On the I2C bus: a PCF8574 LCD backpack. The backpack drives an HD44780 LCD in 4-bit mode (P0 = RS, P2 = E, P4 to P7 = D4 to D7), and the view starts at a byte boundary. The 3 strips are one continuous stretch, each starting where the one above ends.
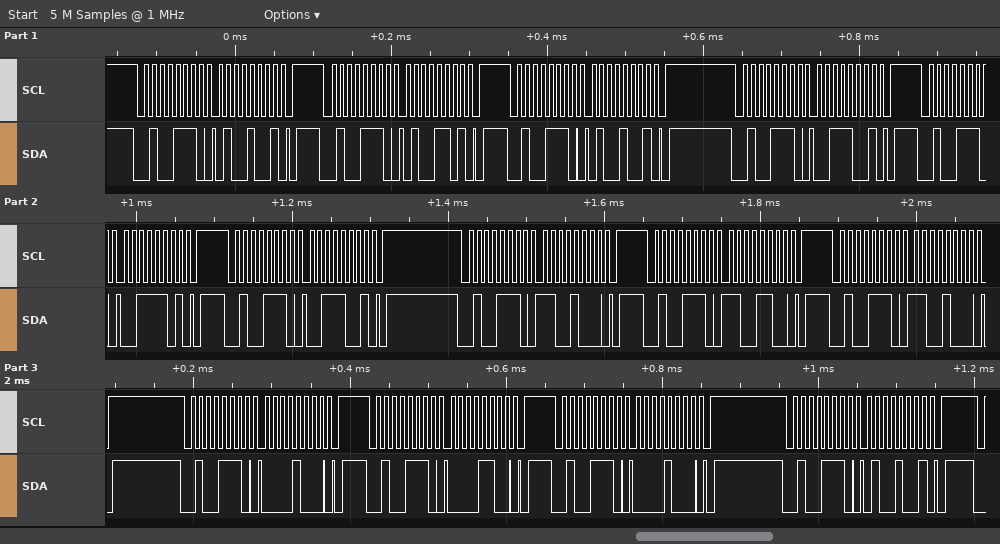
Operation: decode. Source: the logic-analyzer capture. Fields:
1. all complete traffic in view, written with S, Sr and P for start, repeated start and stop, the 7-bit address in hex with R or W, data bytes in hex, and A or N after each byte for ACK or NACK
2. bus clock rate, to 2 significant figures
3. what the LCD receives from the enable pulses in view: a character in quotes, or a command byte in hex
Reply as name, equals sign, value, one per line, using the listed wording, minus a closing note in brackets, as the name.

all complete traffic in view, written with S, Sr and P for start, repeated start and stop, the 7-bit address in hex with R or W, data bytes in hex, and A or N after each byte for ACK or NACK = S 27W A 49 A P S 27W A 4D A P S 27W A 49 A P S 27W A 39 A P S 27W A 3D A P S 27W A 39 A P S 27W A C8 A P S 27W A CC A P S 27W A C8 A P S 27W A 08 A P S 27W A 0C A P S 27W A 08 A P S 27W A 49 A P
bus clock rate, to 2 significant figures = 100 kHz
what the LCD receives from the enable pulses in view: a character in quotes, or a command byte in hex = 'C' 0xC0
